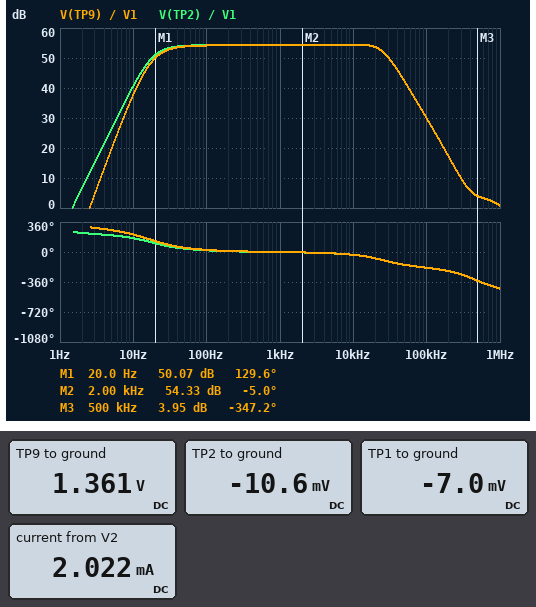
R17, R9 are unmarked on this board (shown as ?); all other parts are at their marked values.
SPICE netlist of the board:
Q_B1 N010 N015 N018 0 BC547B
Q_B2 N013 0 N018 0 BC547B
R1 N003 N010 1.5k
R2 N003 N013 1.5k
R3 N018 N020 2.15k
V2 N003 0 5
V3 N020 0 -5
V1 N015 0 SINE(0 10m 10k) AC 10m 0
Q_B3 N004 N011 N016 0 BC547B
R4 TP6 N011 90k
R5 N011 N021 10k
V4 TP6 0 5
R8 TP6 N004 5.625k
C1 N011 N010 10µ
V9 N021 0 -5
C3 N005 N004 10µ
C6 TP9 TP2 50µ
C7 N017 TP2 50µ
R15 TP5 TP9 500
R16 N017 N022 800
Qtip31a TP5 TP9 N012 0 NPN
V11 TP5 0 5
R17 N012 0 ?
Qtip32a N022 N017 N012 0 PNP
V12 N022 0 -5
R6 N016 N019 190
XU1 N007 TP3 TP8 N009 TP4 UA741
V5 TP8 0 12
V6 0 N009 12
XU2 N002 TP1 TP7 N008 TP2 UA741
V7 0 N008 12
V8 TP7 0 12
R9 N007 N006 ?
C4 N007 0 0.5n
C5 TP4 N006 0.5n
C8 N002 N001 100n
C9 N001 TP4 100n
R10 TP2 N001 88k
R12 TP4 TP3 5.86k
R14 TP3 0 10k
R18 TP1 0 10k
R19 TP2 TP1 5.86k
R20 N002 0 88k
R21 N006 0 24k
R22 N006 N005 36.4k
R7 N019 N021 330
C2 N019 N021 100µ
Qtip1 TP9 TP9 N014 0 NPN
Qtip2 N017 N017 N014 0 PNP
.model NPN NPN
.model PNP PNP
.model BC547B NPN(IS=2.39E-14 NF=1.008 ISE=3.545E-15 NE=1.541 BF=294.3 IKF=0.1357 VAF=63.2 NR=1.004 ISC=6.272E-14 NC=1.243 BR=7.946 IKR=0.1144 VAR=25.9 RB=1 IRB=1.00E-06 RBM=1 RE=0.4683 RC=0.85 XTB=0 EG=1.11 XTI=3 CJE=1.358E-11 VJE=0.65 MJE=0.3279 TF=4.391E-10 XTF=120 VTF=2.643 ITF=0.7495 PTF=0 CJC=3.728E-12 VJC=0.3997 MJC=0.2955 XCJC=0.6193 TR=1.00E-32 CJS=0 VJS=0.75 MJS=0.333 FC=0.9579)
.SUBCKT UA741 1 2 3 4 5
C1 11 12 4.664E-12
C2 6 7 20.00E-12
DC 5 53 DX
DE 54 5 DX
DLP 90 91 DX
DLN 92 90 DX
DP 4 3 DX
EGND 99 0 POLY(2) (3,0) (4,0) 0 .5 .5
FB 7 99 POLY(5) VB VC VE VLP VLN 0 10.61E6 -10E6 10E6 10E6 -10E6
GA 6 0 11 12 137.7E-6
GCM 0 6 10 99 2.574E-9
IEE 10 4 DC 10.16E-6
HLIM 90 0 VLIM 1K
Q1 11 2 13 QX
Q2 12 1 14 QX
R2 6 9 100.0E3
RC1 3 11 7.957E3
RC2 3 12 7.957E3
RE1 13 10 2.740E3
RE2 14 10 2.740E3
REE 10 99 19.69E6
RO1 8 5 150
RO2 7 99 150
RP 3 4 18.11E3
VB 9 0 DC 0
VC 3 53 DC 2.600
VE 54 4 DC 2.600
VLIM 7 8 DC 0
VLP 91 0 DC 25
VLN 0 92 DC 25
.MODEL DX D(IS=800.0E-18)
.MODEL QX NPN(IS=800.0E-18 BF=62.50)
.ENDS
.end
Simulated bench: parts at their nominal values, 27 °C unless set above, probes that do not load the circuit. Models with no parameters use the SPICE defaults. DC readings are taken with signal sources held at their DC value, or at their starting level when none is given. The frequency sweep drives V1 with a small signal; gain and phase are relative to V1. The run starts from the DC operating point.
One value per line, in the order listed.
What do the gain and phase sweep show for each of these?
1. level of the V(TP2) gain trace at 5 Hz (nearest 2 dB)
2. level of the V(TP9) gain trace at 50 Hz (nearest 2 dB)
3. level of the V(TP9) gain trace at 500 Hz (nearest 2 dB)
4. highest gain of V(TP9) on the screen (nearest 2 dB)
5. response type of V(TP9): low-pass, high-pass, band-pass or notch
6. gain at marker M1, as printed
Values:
26 dB
54 dB
54 dB
54 dB
band-pass
50.07 dB
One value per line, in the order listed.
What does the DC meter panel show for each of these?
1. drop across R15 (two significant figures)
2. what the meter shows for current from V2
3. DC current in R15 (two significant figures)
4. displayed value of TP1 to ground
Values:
3.6 V
2.022 mA
7.3 mA
-7.0 mV
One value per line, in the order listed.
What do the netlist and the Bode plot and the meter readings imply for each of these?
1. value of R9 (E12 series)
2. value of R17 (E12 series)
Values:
10 kΩ
3.3 Ω
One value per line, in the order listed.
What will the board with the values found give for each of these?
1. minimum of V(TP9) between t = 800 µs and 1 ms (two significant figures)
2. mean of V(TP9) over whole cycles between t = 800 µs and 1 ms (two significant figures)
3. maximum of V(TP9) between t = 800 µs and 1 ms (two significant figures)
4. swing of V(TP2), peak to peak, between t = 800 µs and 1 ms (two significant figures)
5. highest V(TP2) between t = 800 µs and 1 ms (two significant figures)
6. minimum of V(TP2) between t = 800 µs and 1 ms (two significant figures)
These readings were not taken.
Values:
-2.8 V
1.1 V
5.1 V
7.9 V
3.7 V
-4.2 V
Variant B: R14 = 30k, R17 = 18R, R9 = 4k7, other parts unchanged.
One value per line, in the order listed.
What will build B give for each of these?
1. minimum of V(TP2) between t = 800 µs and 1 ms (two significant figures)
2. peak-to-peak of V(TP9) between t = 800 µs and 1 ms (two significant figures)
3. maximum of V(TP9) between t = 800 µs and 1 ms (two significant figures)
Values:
-3.8 V
6.4 V
4.2 V
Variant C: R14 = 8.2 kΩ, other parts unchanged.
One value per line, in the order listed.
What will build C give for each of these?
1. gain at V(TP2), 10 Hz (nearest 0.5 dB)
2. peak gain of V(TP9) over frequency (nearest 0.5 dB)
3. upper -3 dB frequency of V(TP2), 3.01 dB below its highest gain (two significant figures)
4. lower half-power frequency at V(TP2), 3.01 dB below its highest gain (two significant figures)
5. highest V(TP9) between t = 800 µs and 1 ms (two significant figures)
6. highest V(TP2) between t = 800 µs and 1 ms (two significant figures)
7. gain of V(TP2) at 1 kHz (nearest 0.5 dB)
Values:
41.5 dB
55.5 dB
28 kHz
23 Hz
5.4 V
4.1 V
55.0 dB
